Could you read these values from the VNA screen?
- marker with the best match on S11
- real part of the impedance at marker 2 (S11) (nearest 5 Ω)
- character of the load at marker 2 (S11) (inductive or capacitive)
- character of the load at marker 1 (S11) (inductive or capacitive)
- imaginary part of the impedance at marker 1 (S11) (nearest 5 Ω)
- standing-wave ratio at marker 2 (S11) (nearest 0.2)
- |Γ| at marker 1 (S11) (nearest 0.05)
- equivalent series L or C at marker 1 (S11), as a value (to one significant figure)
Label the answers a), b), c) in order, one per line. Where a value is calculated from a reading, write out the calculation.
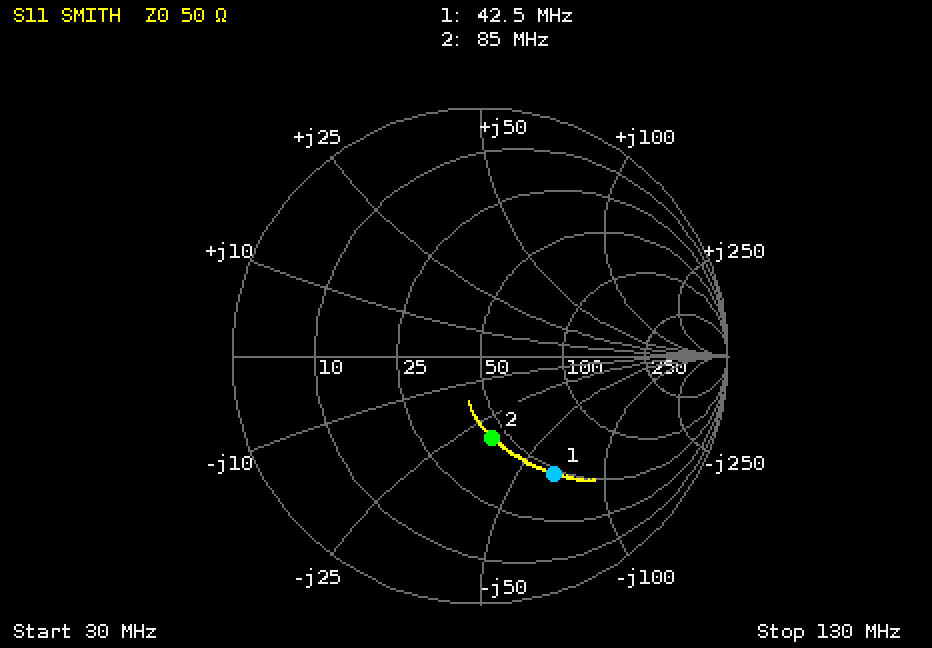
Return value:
a) marker 2
b) 45 Ω
c) capacitive
d) capacitive
e) -65 Ω
f) 2.0
g) 0.55
h) C = 1/(2π × 42.5 MHz × 65 Ω) ≈ 57.6 pF, so 60 pF to one significant figure
